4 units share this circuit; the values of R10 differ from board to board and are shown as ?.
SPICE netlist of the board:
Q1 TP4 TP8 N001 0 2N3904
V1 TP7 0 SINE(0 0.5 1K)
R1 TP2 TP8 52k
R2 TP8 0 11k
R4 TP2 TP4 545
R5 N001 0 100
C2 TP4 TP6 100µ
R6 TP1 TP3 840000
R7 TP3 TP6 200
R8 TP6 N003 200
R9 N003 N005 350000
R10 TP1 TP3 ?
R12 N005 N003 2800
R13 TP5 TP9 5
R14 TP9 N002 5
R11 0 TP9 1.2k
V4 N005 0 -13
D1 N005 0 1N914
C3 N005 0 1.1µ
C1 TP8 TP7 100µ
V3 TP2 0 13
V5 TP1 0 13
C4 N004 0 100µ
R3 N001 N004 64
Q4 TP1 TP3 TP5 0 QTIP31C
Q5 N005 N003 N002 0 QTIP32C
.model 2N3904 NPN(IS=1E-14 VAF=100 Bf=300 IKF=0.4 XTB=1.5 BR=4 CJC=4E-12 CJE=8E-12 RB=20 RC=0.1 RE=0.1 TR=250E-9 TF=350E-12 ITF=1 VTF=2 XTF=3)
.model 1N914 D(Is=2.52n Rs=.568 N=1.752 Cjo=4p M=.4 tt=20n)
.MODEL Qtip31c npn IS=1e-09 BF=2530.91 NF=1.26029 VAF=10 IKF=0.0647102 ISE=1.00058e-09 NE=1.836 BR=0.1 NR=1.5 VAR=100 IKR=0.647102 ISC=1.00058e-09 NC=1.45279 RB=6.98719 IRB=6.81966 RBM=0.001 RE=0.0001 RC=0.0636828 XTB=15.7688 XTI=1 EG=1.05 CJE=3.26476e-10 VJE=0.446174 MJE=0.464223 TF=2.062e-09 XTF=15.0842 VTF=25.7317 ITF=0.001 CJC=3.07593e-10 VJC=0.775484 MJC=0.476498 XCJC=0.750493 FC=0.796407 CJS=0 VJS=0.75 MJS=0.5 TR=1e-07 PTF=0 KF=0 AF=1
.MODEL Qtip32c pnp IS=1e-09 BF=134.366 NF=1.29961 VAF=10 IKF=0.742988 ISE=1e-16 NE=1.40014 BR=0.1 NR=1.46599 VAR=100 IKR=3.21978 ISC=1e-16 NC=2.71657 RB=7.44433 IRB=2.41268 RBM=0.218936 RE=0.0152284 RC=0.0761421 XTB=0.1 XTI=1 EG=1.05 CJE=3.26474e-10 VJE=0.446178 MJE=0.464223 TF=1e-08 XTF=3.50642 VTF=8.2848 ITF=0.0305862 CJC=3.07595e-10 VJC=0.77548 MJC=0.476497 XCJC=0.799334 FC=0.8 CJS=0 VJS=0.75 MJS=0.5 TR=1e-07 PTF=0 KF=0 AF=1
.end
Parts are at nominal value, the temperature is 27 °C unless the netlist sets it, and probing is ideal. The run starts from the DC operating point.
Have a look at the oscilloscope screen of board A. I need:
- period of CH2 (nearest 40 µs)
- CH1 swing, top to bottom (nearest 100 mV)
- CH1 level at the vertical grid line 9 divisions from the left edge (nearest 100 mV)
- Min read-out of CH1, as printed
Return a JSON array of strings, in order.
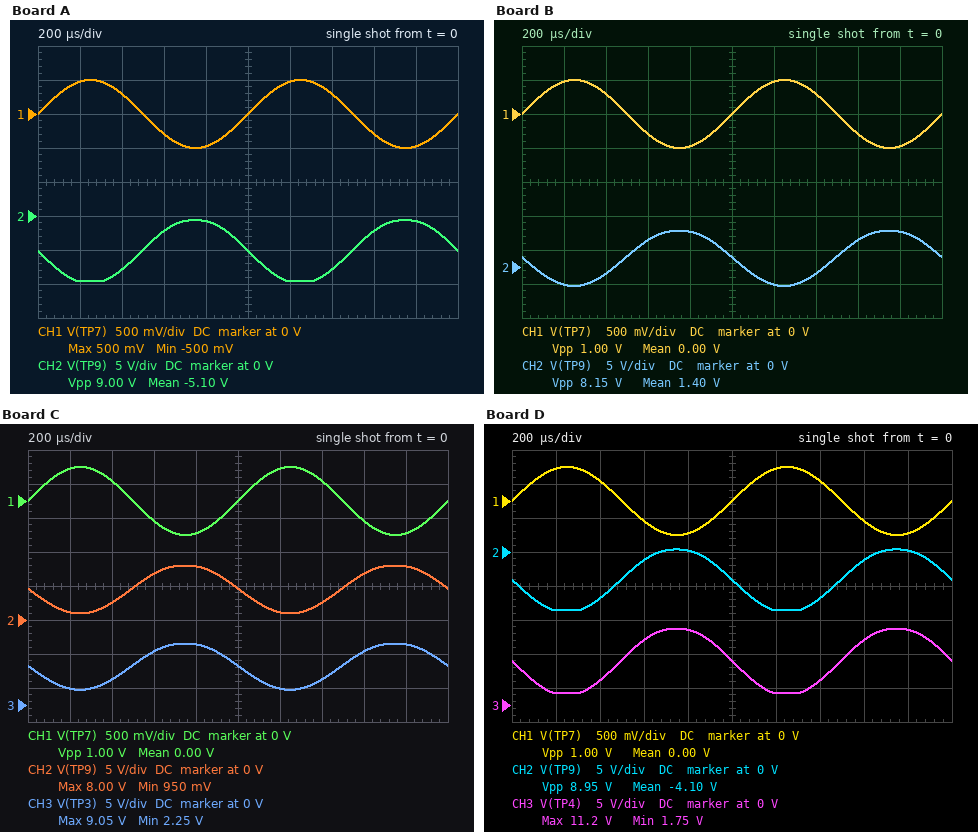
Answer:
["1.00 ms", "1.0 V", "-500 mV", "-500 mV"]
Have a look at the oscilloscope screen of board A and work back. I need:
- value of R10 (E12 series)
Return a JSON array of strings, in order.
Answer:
["6.8 kΩ"]
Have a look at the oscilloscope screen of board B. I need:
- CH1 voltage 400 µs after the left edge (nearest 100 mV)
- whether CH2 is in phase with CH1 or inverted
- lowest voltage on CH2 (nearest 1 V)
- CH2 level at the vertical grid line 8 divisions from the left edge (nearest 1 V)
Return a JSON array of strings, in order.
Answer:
["300 mV", "inverted", "-3 V", "4 V"]
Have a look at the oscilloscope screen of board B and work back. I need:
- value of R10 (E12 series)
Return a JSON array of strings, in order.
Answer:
["2.2 kΩ"]
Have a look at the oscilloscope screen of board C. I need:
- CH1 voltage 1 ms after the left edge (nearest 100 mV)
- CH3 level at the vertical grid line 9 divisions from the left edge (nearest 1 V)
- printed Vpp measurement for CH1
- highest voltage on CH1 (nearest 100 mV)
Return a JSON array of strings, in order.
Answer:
["0 V", "9 V", "1.00 V", "500 mV"]
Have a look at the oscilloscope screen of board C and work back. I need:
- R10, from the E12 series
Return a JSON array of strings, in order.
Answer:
["1.2 kΩ"]
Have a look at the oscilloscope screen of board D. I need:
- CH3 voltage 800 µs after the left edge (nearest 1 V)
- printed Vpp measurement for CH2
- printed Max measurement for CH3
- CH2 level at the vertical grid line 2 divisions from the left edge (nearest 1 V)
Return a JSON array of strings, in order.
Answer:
["11 V", "8.95 V", "11.2 V", "-7 V"]
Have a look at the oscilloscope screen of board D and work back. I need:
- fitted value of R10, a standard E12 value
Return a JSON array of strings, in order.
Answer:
["5.6 kΩ"]
